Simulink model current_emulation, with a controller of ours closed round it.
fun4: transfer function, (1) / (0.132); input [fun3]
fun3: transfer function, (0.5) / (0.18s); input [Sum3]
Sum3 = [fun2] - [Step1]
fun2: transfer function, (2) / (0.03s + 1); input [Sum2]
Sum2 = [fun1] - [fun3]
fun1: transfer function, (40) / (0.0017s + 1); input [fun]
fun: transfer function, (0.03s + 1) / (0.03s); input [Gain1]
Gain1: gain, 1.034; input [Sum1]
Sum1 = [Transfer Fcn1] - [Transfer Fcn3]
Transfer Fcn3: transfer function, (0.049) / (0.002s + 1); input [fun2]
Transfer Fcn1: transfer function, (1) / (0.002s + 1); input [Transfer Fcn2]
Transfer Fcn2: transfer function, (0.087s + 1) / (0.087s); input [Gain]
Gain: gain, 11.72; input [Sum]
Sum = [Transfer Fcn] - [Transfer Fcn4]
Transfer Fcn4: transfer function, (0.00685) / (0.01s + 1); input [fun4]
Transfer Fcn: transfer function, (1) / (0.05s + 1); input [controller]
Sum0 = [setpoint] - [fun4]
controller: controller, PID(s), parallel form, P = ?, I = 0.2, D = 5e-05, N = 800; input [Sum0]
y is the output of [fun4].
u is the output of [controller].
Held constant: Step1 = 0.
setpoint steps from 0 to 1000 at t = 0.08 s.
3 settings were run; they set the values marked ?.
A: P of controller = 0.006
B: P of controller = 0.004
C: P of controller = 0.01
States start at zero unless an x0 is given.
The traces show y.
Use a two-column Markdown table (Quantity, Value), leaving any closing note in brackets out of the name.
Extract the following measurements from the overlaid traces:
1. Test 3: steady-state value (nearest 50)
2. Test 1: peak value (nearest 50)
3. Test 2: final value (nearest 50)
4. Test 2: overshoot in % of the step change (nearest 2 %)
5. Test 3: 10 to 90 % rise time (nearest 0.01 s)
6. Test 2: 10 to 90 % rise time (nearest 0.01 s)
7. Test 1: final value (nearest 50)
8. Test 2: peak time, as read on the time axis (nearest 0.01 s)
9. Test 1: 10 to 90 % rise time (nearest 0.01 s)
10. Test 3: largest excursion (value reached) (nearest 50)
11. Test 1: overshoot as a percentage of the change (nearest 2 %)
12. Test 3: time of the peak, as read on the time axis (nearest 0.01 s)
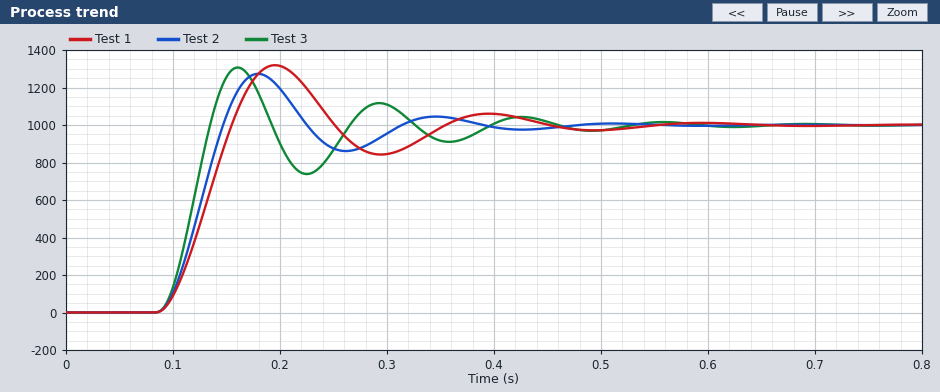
| Quantity | Value |
|---|---|
| Test 3: steady-state value | 1000 |
| Test 1: peak value | 1300 |
| Test 2: final value | 1000 |
| Test 2: overshoot in % of the step change | 28 % |
| Test 3: 10 to 90 % rise time | 0.03 s |
| Test 2: 10 to 90 % rise time | 0.04 s |
| Test 1: final value | 1000 |
| Test 2: peak time, as read on the time axis | 0.18 s |
| Test 1: 10 to 90 % rise time | 0.05 s |
| Test 3: largest excursion (value reached) | 1300 |
| Test 1: overshoot as a percentage of the change | 32 % |
| Test 3: time of the peak, as read on the time axis | 0.16 s |
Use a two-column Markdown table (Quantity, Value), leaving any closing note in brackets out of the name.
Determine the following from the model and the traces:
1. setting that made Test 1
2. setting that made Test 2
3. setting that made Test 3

| Quantity | Value |
|---|---|
| setting that made Test 1 | B |
| setting that made Test 2 | A |
| setting that made Test 3 | C |
